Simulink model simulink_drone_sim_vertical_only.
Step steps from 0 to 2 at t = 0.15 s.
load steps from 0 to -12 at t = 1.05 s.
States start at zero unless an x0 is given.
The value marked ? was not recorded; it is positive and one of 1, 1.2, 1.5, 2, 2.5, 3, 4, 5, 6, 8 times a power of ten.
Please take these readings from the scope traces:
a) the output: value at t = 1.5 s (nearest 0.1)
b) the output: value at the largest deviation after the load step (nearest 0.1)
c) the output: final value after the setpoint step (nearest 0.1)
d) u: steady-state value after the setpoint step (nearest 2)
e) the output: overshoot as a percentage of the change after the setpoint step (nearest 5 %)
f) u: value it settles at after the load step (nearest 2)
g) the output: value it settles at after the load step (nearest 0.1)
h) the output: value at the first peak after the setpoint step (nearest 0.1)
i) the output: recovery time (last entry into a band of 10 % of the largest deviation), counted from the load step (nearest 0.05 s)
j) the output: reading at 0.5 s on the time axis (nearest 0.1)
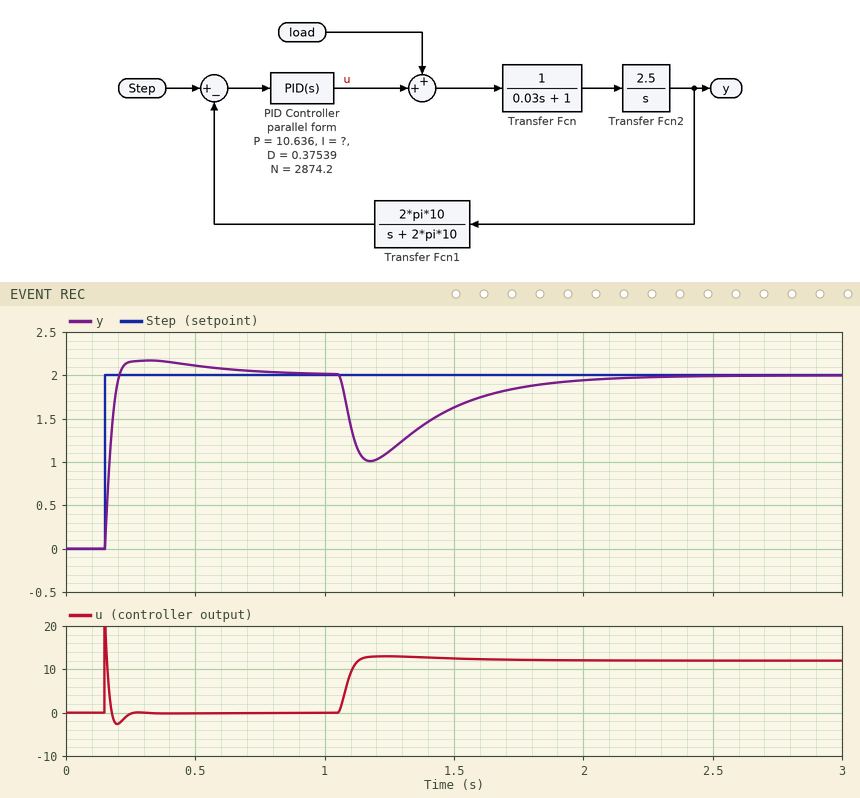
1.6
1.0
2.0
0
10 %
12
2.0
2.2
0.80 s
2.1
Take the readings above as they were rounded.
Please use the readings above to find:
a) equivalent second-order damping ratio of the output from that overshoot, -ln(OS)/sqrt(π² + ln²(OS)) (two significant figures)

0.59
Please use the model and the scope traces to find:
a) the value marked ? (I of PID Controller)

30
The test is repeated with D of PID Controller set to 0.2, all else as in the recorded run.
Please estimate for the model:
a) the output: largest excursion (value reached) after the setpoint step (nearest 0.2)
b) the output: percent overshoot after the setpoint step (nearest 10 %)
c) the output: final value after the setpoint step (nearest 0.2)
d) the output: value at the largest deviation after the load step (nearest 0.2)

2.4
20 %
2.0
0.8
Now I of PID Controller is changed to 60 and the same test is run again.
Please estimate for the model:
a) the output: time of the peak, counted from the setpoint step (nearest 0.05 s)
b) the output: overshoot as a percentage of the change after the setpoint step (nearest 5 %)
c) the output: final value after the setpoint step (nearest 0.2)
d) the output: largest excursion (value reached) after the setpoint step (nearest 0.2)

0.15 s
15 %
2.0
2.4
